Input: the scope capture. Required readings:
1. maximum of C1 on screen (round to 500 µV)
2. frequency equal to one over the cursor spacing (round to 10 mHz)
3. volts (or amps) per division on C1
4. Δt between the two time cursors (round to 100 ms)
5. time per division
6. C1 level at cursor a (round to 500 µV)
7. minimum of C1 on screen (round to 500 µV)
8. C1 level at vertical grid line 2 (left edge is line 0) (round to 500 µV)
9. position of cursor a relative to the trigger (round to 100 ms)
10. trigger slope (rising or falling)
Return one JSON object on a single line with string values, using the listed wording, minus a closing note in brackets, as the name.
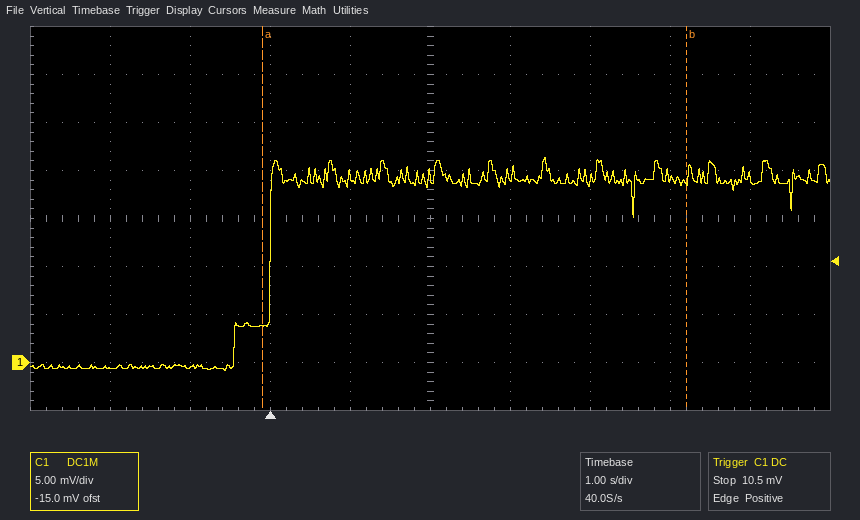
{"maximum of C1 on screen": "21.5 mV", "frequency equal to one over the cursor spacing": "190 mHz", "volts (or amps) per division on C1": "5 mV", "Δt between the two time cursors": "5.3 s", "time per division": "1 s", "C1 level at cursor a": "4.0 mV", "minimum of C1 on screen": "-1.0 mV", "C1 level at vertical grid line 2 (left edge is line 0)": "-500 µV", "position of cursor a relative to the trigger": "-100 ms", "trigger slope": "rising"}
